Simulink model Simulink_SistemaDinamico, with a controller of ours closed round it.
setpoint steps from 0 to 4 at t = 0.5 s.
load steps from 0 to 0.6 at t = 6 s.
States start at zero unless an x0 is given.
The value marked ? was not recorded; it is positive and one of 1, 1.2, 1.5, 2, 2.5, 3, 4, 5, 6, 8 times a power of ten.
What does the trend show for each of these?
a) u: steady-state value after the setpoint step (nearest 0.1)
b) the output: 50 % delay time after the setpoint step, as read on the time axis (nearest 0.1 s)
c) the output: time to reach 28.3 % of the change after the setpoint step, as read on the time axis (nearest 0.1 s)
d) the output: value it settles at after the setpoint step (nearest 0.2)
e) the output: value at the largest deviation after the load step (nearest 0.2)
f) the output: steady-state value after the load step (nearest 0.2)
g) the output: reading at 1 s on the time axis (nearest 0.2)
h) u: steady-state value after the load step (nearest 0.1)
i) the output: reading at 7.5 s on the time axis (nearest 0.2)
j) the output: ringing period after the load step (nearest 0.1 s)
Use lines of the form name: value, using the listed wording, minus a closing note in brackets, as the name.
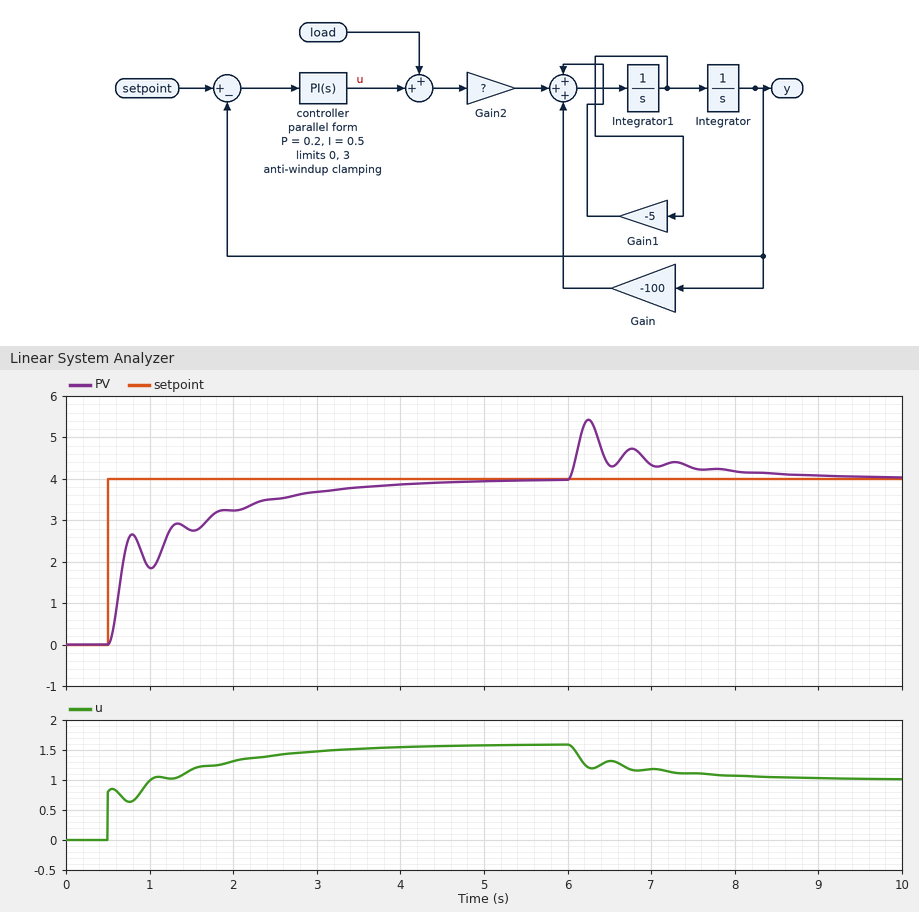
u: steady-state value after the setpoint step: 1.6
the output: 50 % delay time after the setpoint step, as read on the time axis: 0.7 s
the output: time to reach 28.3 % of the change after the setpoint step, as read on the time axis: 0.6 s
the output: value it settles at after the setpoint step: 4.0
the output: value at the largest deviation after the load step: 5.4
the output: steady-state value after the load step: 4.0
the output: reading at 1 s on the time axis: 1.8
u: steady-state value after the load step: 1.0
the output: reading at 7.5 s on the time axis: 4.2
the output: ringing period after the load step: 0.5 s
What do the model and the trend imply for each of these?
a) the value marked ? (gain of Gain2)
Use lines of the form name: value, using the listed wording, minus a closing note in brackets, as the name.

the value marked ?: 250
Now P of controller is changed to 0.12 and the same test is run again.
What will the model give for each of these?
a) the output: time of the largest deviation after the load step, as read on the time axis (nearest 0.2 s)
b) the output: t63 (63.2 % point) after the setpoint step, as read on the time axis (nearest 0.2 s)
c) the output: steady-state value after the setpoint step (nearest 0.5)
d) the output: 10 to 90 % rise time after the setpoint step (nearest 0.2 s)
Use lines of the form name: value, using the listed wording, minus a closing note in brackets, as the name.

the output: time of the largest deviation after the load step, as read on the time axis: 6.2 s
the output: t63 (63.2 % point) after the setpoint step, as read on the time axis: 1.2 s
the output: steady-state value after the setpoint step: 4.0
the output: 10 to 90 % rise time after the setpoint step: 2.0 s
